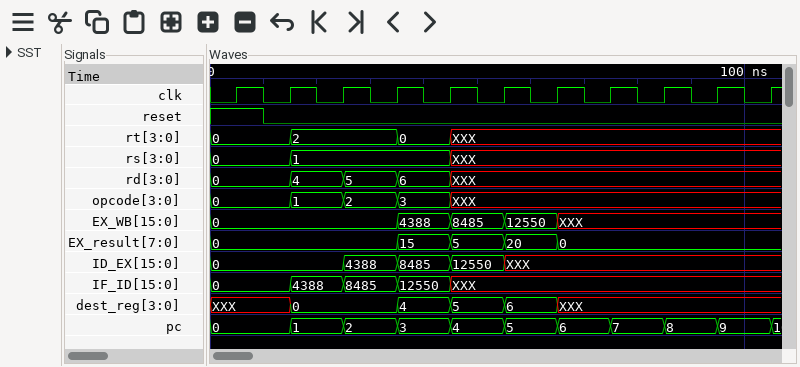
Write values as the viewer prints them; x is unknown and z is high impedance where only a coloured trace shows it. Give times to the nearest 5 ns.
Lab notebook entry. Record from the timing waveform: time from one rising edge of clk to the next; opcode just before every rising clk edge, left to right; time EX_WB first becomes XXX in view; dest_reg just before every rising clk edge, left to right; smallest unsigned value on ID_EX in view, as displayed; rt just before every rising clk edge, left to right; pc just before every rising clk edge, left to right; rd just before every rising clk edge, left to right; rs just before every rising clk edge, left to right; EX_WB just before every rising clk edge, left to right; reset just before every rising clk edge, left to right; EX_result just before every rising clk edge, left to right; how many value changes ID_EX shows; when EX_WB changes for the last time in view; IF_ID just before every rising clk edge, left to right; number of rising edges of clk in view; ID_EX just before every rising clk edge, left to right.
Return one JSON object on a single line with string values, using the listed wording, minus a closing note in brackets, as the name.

{"time from one rising edge of clk to the next": "10 ns", "opcode just before every rising clk edge, left to right": "0, 0, 1, 2, 3, XXX, XXX, XXX, XXX, XXX, XXX", "time EX_WB first becomes XXX in view": "65 ns", "dest_reg just before every rising clk edge, left to right": "XXX, XXX, 0, 0, 4, 5, 6, XXX, XXX, XXX, XXX", "smallest unsigned value on ID_EX in view, as displayed": "0", "rt just before every rising clk edge, left to right": "0, 0, 2, 2, 0, XXX, XXX, XXX, XXX, XXX, XXX", "pc just before every rising clk edge, left to right": "0, 0, 1, 2, 3, 4, 5, 6, 7, 8, 9", "rd just before every rising clk edge, left to right": "0, 0, 4, 5, 6, XXX, XXX, XXX, XXX, XXX, XXX", "rs just before every rising clk edge, left to right": "0, 0, 1, 1, 1, XXX, XXX, XXX, XXX, XXX, XXX", "EX_WB just before every rising clk edge, left to right": "0, 0, 0, 0, 4388, 8485, 12550, XXX, XXX, XXX, XXX", "reset just before every rising clk edge, left to right": "1 0 0 0 0 0 0 0 0 0 0", "EX_result just before every rising clk edge, left to right": "0, 0, 0, 0, 15, 5, 20, 0, 0, 0, 0", "how many value changes ID_EX shows": "4", "when EX_WB changes for the last time in view": "65 ns", "IF_ID just before every rising clk edge, left to right": "0, 0, 4388, 8485, 12550, XXX, XXX, XXX, XXX, XXX, XXX", "number of rising edges of clk in view": "11", "ID_EX just before every rising clk edge, left to right": "0, 0, 0, 4388, 8485, 12550, XXX, XXX, XXX, XXX, XXX"}
